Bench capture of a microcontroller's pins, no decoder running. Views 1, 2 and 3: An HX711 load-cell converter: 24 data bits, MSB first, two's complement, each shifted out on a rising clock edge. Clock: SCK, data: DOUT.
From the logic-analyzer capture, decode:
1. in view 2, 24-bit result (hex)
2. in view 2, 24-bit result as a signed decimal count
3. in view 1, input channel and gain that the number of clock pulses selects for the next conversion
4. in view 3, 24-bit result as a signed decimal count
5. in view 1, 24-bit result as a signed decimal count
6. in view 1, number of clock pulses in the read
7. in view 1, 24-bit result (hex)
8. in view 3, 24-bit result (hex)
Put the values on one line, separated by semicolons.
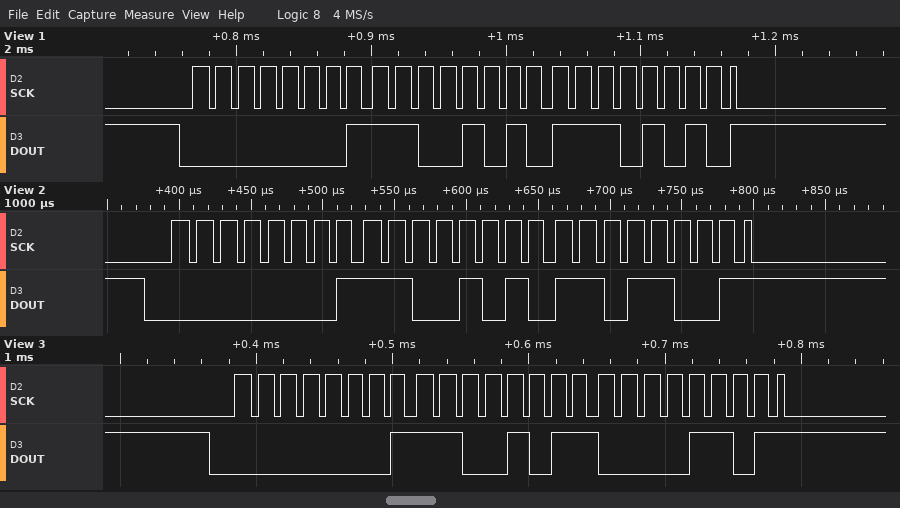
0x01CAD9; 117465; channel A, gain 128; 117517; 117482; 25; 0x01CAEA; 0x01CB0D
